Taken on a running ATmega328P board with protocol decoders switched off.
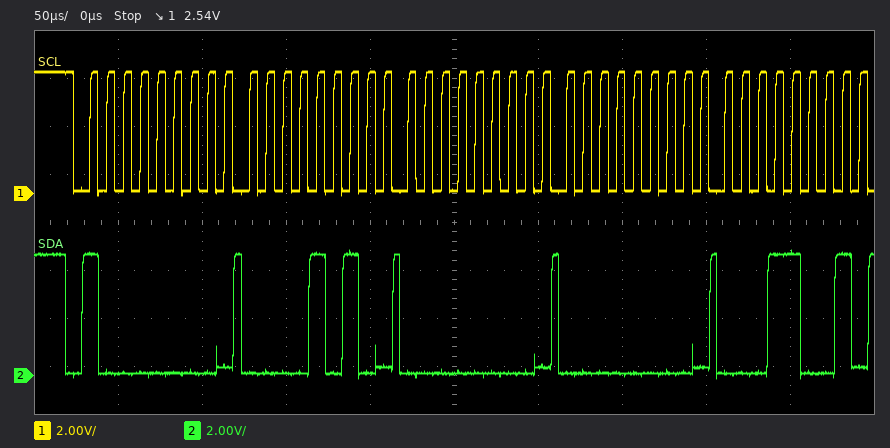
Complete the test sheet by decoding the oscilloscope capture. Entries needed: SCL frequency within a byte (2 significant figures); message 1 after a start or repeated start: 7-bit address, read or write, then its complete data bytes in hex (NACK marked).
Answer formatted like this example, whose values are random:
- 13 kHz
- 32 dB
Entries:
- 100 kHz
- 0x40 write: 0A 00 00 19
